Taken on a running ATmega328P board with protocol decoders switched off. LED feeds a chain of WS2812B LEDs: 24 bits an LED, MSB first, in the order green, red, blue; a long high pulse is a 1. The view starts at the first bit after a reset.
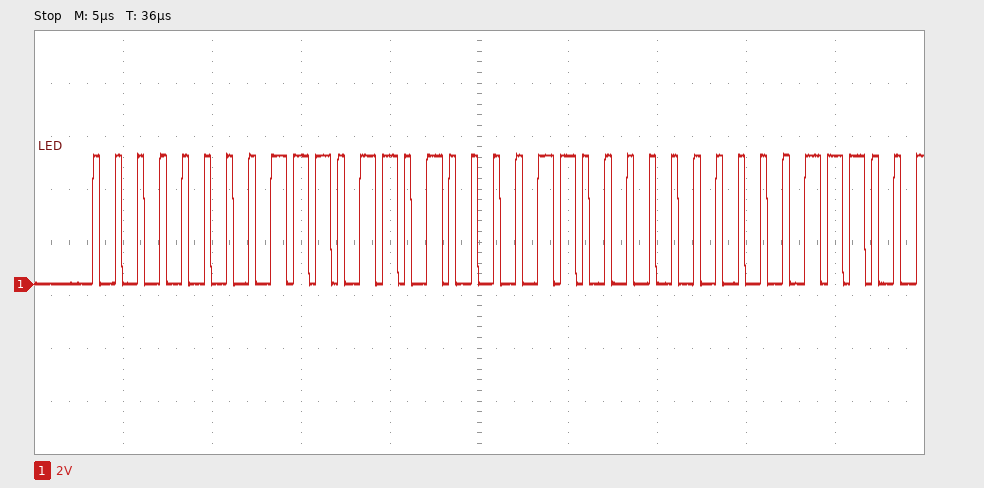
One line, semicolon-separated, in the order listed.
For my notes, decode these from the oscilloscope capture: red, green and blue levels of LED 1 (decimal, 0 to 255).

237, 0, 12
